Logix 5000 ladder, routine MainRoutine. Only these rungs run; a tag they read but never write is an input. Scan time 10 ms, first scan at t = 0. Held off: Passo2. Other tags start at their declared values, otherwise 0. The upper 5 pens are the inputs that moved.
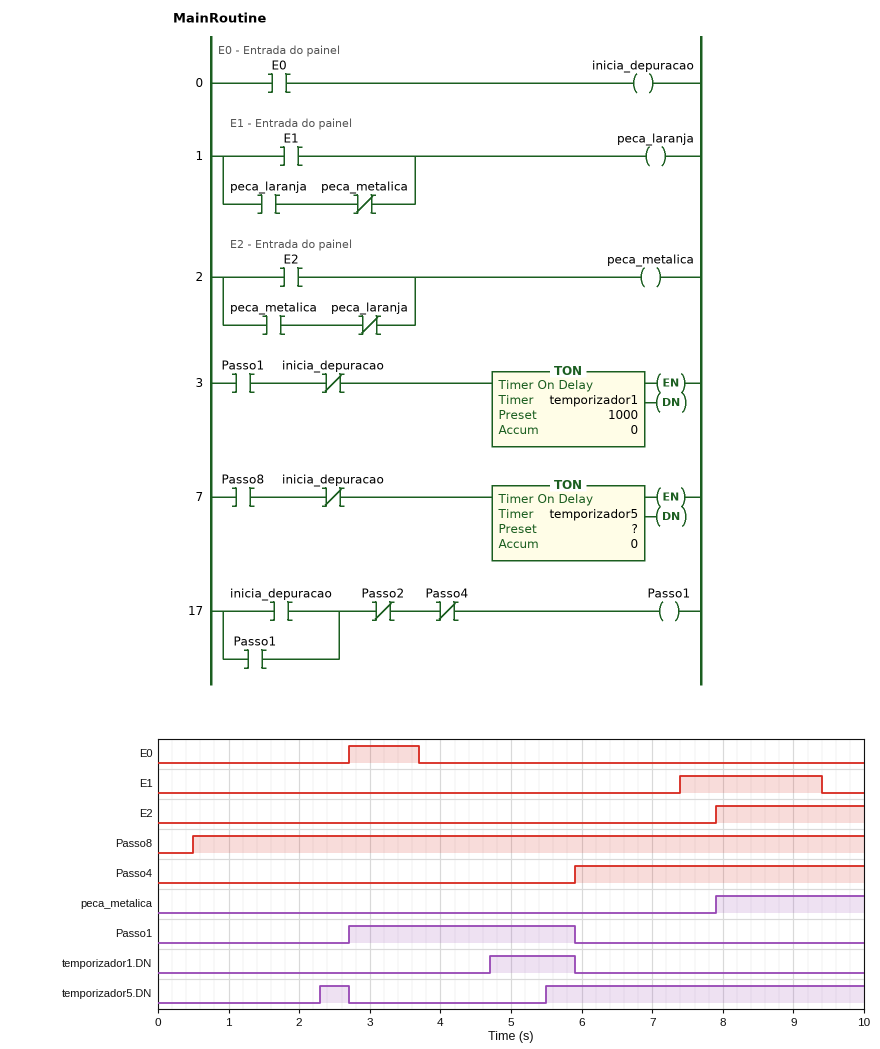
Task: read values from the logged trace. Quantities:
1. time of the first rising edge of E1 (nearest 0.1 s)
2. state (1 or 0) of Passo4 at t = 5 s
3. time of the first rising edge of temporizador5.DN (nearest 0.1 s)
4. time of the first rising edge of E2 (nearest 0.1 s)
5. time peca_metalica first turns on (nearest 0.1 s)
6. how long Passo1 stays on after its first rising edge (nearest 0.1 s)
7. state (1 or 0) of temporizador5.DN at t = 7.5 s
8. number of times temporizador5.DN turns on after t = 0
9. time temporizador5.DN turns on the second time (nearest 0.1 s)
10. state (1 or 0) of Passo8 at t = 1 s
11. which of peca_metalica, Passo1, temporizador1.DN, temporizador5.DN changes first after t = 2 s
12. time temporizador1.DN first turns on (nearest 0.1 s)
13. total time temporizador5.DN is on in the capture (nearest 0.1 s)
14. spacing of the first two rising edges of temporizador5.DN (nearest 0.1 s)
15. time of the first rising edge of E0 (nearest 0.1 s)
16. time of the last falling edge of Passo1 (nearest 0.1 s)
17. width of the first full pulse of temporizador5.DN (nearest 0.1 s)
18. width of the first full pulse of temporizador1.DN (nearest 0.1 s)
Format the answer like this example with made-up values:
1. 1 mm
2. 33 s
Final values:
1. 7.4 s
2. 0
3. 2.3 s
4. 7.9 s
5. 7.9 s
6. 3.2 s
7. 1
8. 2
9. 5.5 s
10. 1
11. temporizador5.DN
12. 4.7 s
13. 4.9 s
14. 3.2 s
15. 2.7 s
16. 5.9 s
17. 0.4 s
18. 1.2 s
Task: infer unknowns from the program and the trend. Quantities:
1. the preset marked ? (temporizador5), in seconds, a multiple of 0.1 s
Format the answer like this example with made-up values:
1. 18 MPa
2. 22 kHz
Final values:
1. 1.8 s
